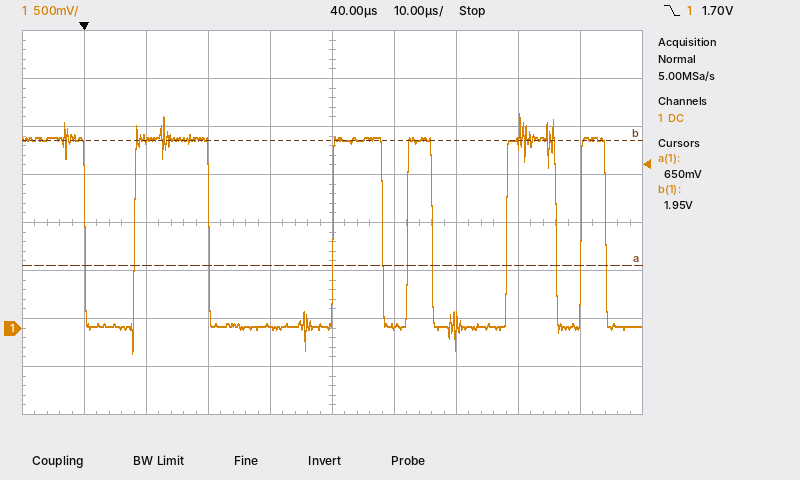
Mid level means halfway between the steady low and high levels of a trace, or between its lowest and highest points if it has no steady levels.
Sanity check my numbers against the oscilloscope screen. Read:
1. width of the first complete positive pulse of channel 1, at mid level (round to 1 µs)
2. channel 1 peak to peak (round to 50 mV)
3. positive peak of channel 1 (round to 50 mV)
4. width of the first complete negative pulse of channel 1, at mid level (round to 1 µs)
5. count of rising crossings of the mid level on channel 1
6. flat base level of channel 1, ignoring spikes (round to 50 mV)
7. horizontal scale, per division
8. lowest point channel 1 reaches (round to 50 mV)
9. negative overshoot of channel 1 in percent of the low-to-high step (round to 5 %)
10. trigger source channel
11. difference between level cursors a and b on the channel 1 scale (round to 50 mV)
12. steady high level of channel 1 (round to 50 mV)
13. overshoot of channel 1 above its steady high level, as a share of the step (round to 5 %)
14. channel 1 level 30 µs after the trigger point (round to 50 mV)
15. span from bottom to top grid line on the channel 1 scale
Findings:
12 µs
2.50 V
2.25 V
8 µs
5
0 mV
10 µs
-250 mV
15 %
channel 1
1.30 V
1.95 V
15 %
0 mV
4 V
